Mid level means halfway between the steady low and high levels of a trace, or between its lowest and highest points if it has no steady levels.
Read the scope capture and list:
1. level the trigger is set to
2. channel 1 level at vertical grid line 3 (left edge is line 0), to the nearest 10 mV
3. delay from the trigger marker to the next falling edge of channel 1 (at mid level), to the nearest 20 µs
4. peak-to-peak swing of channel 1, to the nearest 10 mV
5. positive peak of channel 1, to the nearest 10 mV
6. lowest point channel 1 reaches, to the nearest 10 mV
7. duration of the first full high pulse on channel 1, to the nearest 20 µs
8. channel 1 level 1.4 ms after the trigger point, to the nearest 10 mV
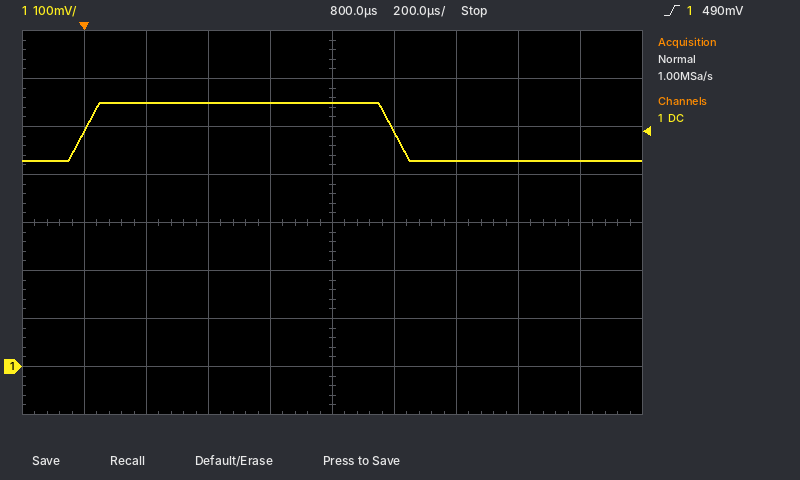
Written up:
490 mV
550 mV
1.00 ms
120 mV
550 mV
430 mV
1.00 ms
430 mV
